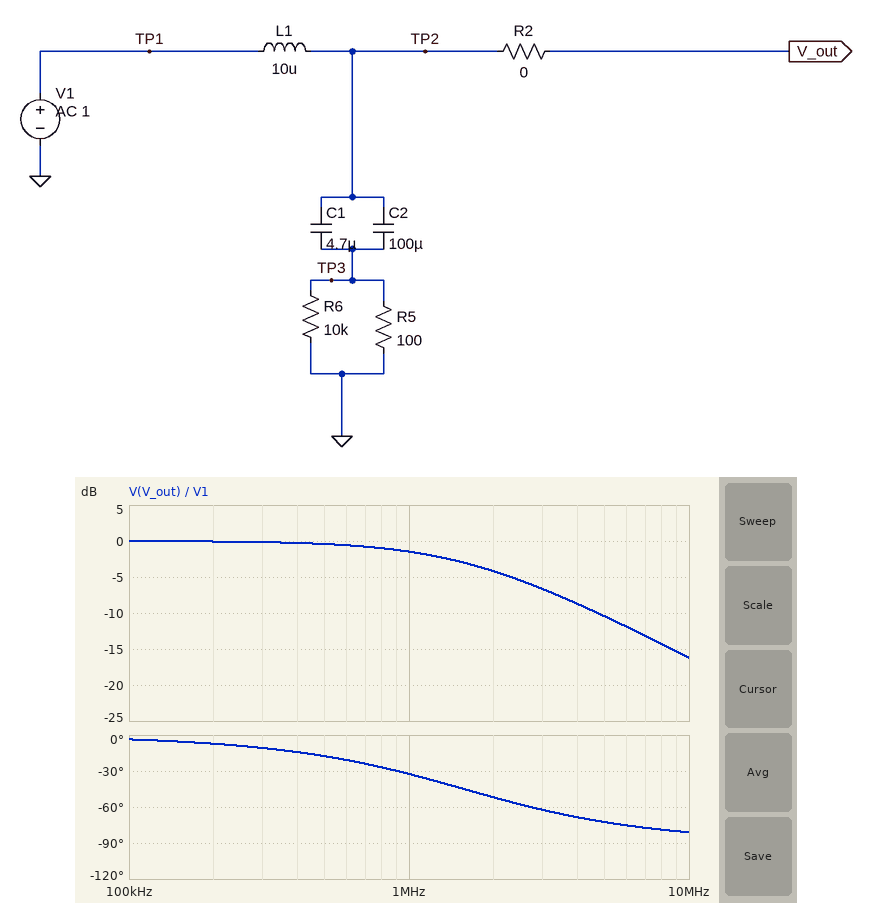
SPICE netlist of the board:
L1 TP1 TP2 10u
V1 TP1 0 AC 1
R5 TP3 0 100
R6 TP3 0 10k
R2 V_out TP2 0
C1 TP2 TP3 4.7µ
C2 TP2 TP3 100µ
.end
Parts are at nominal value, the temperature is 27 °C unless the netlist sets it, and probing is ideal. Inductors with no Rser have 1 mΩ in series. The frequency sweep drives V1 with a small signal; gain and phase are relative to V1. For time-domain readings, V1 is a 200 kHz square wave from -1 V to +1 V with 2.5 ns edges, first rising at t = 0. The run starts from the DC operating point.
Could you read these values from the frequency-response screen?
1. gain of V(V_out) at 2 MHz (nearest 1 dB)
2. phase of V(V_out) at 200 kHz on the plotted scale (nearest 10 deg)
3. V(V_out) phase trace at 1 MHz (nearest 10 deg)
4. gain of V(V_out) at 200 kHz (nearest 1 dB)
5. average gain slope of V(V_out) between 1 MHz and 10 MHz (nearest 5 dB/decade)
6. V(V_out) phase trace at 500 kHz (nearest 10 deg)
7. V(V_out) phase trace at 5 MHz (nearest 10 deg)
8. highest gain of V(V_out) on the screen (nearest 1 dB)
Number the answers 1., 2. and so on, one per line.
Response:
1. -4 dB
2. -10 deg
3. -30 deg
4. 0 dB
5. -15 dB/decade
6. -20 deg
7. -70 deg
8. 0 dB
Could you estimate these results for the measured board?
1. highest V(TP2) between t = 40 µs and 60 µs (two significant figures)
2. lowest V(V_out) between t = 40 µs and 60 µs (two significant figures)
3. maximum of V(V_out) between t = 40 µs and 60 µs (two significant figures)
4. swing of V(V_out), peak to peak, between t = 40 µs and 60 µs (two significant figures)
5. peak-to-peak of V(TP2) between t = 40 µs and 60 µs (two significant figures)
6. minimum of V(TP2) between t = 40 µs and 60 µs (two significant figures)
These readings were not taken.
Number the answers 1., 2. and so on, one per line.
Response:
1. 1.0 V
2. -1.0 V
3. 1.0 V
4. 2.0 V
5. 2.0 V
6. -1.0 V
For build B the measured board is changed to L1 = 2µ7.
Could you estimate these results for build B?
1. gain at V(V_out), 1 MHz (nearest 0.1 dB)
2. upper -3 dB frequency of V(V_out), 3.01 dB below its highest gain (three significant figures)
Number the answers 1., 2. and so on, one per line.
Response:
1. -0.1 dB
2. 5.82 MHz
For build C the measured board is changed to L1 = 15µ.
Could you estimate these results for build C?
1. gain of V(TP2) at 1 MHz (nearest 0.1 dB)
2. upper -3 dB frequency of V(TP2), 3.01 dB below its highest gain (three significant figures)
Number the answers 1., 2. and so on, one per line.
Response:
1. -2.8 dB
2. 1.05 MHz
